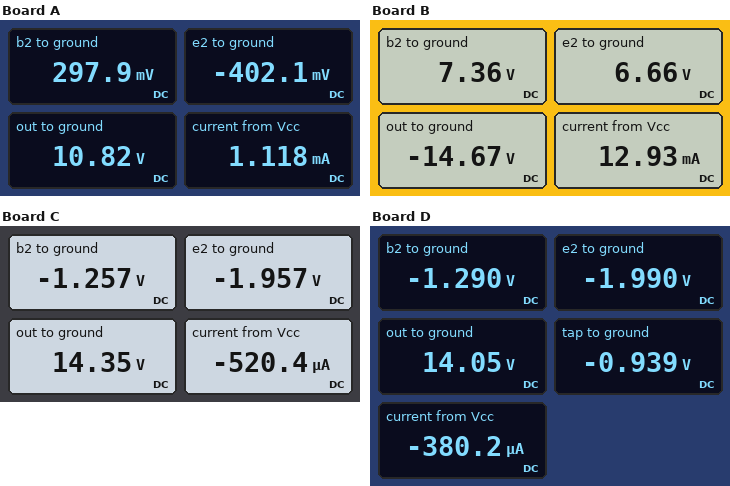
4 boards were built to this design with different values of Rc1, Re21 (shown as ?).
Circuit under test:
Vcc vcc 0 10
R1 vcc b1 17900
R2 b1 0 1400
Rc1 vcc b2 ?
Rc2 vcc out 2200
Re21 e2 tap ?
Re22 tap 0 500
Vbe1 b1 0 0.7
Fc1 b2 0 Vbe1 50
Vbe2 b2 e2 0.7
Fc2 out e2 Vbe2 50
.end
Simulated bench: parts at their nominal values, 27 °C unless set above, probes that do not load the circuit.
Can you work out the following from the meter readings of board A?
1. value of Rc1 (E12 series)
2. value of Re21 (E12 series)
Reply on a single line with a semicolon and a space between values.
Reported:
10 kΩ; 560 Ω
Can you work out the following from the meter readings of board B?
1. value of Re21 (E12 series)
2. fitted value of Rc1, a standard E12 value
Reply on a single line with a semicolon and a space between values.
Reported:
82 Ω; 2.2 kΩ
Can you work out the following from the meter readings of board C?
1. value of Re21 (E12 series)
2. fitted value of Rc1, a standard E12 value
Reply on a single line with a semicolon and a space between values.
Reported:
470 Ω; 12 kΩ
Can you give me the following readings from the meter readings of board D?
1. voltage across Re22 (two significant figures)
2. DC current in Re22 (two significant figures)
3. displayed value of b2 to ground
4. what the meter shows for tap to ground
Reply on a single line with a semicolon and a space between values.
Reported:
940 mV; 1.9 mA; -1.290 V; -0.939 V
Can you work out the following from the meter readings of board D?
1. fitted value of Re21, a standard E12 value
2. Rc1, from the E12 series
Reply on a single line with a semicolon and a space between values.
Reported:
560 Ω; 12 kΩ
